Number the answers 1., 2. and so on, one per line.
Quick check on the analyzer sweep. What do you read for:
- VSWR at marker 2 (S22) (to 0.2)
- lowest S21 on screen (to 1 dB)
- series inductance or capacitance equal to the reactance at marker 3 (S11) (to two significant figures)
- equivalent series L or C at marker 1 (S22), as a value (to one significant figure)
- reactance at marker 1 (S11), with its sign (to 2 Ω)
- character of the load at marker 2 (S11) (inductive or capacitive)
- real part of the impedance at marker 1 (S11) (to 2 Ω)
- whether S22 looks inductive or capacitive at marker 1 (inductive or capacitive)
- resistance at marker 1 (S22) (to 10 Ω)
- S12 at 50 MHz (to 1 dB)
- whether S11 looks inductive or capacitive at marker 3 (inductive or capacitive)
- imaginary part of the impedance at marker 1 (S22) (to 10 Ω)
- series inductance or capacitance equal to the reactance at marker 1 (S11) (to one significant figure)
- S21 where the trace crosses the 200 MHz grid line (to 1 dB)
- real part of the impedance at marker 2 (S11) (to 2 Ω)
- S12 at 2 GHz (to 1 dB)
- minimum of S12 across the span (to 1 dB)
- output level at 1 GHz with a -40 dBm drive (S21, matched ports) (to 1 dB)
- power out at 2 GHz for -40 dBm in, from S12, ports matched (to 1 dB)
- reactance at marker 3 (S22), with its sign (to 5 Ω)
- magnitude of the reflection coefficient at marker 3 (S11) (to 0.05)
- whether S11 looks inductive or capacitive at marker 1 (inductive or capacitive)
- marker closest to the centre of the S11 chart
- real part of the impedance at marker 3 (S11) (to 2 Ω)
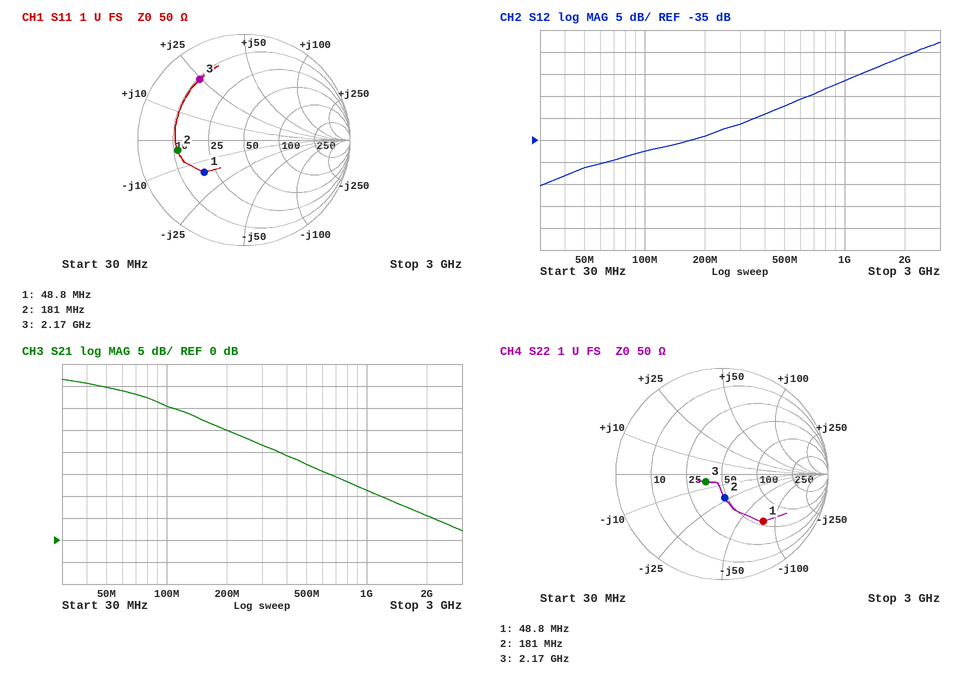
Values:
1. 1.6
2. 2 dB
3. 1.8 nH
4. 40 pF
5. -16 Ω
6. capacitive
7. 20 Ω
8. capacitive
9. 60 Ω
10. -41 dB
11. inductive
12. -80 Ω
13. 200 pF
14. 25 dB
15. 12 Ω
16. -16 dB
17. -45 dB
18. -29 dBm
19. -56 dBm
20. -5 Ω
21. 0.70
22. capacitive
23. marker 1
24. 10 Ω
